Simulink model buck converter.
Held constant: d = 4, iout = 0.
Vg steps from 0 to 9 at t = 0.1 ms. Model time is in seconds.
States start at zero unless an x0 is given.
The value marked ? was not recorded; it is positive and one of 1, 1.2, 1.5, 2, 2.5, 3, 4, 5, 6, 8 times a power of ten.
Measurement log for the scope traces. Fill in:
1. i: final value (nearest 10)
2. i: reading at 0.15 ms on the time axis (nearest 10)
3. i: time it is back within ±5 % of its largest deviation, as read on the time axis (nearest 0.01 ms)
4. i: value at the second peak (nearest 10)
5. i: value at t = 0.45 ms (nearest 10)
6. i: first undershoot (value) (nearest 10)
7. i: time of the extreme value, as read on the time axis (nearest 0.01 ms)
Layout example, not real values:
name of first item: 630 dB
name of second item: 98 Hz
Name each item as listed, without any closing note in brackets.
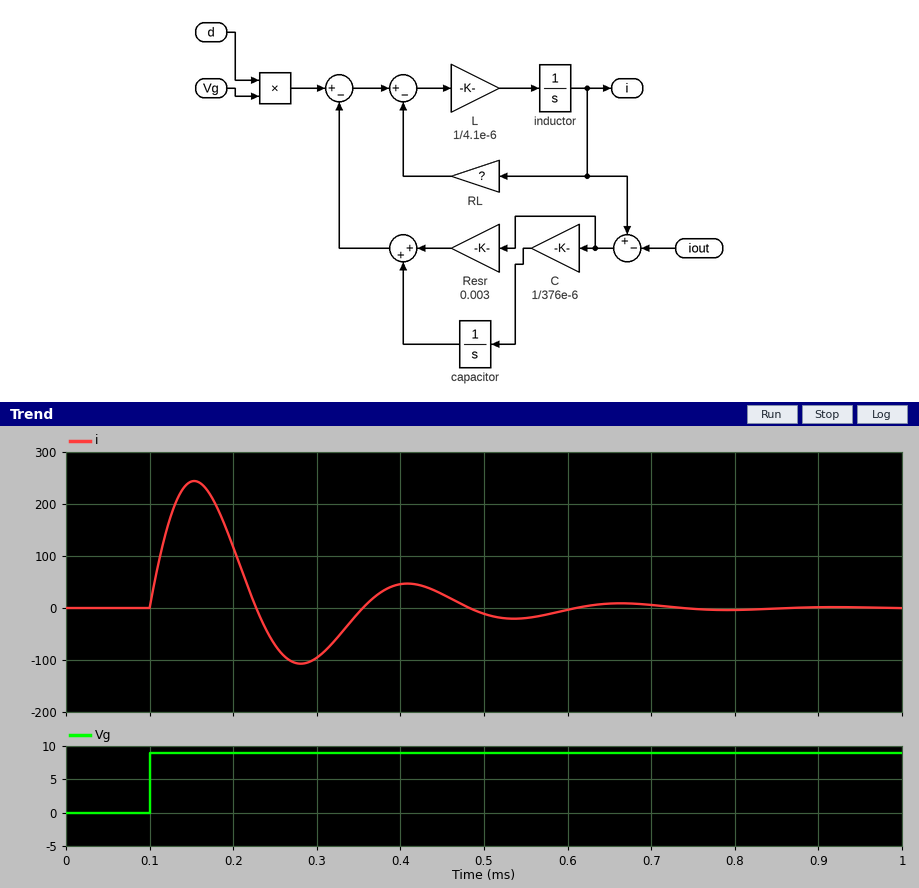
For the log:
i: final value: 0
i: reading at 0.15 ms on the time axis: 240
i: time it is back within ±5 % of its largest deviation, as read on the time axis: 0.58 ms
i: value at the second peak: 50
i: value at t = 0.45 ms: 30
i: first undershoot (value): -110
i: time of the extreme value, as read on the time axis: 0.15 ms
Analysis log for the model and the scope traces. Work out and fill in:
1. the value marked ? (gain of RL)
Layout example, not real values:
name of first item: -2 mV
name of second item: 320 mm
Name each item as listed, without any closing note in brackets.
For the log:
the value marked ?: 0.05
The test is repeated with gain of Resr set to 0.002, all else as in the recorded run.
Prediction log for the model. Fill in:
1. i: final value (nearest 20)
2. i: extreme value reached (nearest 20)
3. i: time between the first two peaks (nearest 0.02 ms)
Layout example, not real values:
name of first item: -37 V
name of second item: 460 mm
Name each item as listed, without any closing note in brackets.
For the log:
i: final value: 0
i: extreme value reached: 240
i: time between the first two peaks: 0.26 ms
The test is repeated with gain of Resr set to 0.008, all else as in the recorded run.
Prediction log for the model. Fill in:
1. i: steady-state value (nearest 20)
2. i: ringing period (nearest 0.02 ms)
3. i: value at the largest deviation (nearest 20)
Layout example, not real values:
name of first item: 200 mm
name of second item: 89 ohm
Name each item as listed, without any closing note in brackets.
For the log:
i: steady-state value: 0
i: ringing period: 0.26 ms
i: value at the largest deviation: 240
